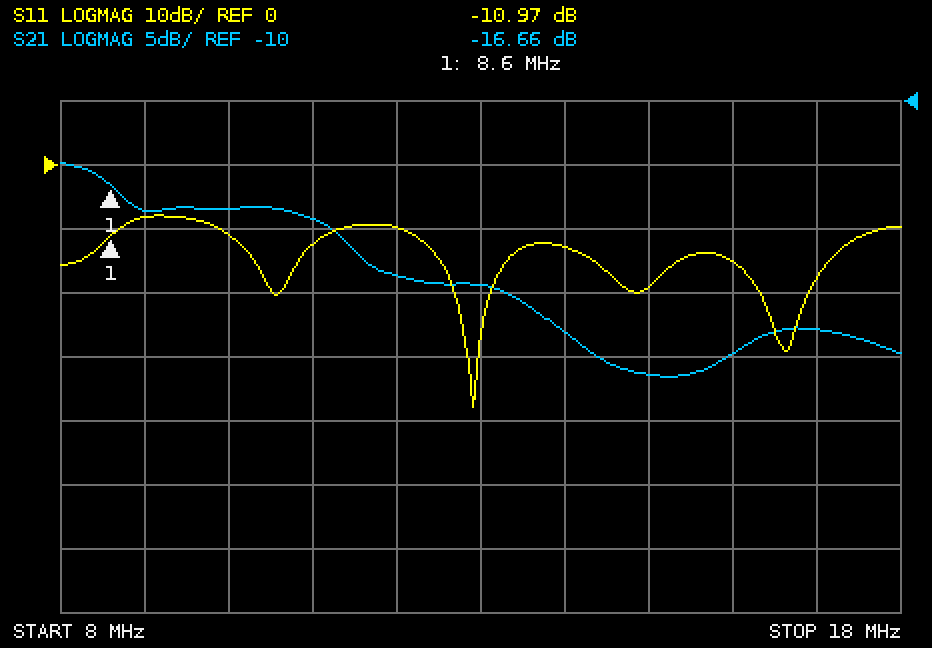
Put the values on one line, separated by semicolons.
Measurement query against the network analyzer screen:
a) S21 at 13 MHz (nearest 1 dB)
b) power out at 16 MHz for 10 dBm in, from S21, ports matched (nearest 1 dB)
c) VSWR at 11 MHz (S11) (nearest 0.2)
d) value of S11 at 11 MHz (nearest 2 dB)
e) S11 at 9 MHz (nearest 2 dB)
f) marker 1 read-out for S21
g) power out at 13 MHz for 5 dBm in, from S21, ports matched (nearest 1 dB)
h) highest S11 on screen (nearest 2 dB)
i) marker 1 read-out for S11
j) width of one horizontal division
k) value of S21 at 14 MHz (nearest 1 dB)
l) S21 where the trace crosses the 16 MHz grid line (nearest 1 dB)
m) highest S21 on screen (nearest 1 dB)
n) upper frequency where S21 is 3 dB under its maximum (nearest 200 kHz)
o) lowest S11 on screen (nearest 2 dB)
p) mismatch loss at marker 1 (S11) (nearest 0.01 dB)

-24 dB; -20 dBm; 1.6; -12 dB; -8 dB; -16.66 dB; -19 dBm; -8 dB; -10.97 dB; 1 MHz; -28 dB; -30 dB; -15 dB; 8.8 MHz; -38 dB; 0.36 dB
